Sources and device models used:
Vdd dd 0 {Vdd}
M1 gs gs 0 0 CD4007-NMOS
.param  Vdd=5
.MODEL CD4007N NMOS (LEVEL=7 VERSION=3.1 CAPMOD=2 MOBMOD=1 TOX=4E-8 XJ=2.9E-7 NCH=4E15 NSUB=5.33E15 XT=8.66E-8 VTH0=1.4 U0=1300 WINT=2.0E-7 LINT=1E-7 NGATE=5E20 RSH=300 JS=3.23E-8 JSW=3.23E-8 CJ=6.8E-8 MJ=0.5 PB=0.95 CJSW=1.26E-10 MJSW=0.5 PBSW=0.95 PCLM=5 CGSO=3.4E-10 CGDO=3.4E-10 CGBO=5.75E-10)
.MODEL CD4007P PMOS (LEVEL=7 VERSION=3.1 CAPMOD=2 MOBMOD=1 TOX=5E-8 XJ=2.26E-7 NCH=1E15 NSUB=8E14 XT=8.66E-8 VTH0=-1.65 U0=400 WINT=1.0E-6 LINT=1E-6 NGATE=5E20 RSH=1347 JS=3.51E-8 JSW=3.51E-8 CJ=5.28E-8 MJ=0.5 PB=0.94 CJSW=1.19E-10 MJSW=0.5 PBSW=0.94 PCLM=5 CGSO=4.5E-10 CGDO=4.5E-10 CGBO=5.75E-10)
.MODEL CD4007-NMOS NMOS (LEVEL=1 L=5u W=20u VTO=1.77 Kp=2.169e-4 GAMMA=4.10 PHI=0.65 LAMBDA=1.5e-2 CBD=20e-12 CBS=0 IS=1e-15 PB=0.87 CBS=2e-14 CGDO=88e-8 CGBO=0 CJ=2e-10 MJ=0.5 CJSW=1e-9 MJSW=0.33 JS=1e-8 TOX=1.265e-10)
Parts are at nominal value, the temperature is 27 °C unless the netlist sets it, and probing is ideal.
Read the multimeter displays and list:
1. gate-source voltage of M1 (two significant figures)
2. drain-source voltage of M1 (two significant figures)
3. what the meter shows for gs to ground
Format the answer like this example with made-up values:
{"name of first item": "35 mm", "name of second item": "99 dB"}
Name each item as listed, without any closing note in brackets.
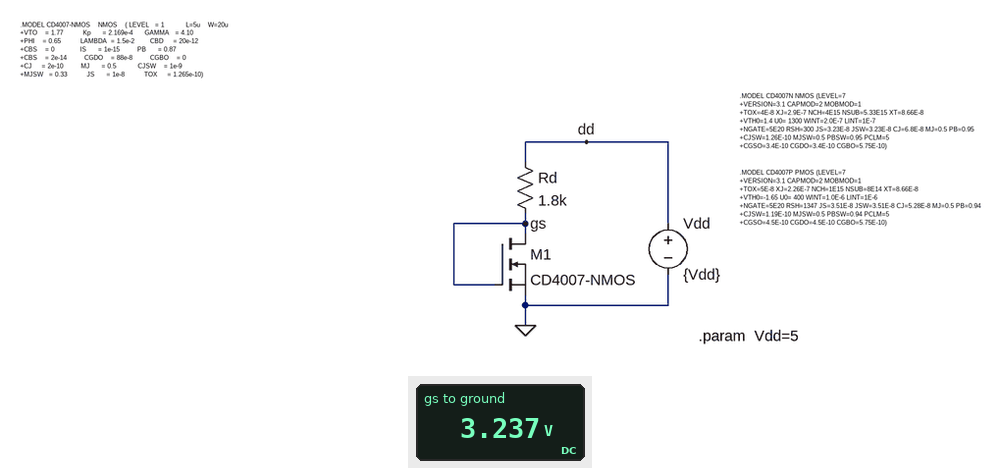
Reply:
{"gate-source voltage of M1": "3.2 V", "drain-source voltage of M1": "3.2 V", "what the meter shows for gs to ground": "3.237 V"}
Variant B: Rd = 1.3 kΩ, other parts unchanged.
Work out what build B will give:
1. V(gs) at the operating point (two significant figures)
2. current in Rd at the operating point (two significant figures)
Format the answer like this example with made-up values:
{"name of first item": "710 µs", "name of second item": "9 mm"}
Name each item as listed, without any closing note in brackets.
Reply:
{"V(gs) at the operating point": "3.4 V", "current in Rd at the operating point": "1.2 mA"}
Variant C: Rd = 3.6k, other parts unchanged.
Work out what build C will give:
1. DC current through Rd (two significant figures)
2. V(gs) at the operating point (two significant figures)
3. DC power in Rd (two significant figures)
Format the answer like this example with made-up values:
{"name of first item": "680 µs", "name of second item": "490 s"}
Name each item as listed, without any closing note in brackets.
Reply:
{"DC current through Rd": "580 µA", "V(gs) at the operating point": "2.9 V", "DC power in Rd": "1.2 mW"}
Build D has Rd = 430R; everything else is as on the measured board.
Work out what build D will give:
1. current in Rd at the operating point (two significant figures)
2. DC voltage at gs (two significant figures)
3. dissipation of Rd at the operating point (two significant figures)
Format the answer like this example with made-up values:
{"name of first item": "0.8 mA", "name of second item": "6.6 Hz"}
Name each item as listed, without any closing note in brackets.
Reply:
{"current in Rd at the operating point": "2.3 mA", "DC voltage at gs": "4.0 V", "dissipation of Rd at the operating point": "2.3 mW"}
